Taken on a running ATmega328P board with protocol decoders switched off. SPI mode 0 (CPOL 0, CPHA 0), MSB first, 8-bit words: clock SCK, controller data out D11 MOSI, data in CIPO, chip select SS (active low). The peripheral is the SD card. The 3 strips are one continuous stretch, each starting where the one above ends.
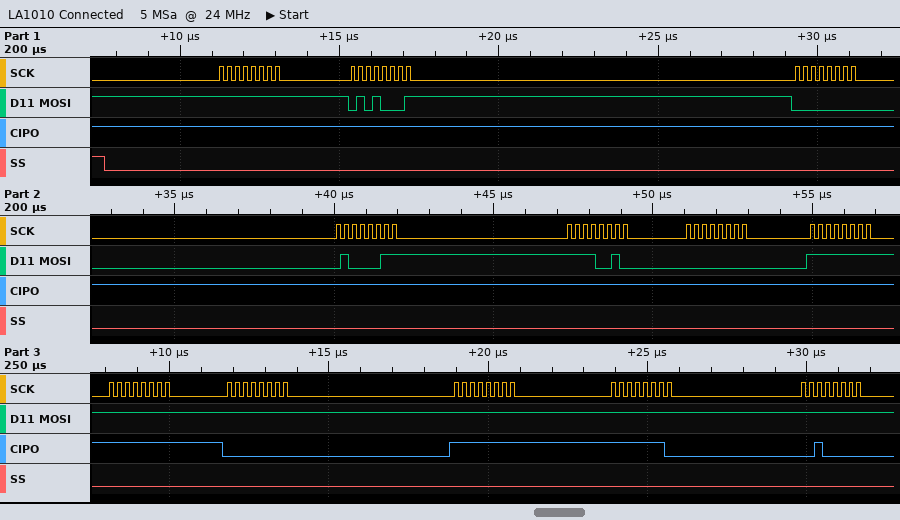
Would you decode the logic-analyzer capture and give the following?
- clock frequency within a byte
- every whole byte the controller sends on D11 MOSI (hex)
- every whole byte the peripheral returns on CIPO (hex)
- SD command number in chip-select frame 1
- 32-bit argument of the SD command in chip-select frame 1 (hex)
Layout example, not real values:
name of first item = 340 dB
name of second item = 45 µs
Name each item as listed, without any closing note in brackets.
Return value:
clock frequency within a byte = 4 MHz
every whole byte the controller sends on D11 MOSI = FF 51 00 43 F2 00 FF FF FF FF FF FF
every whole byte the peripheral returns on CIPO = FF FF FF FF FF FF FF FF 00 FF FE 20
SD command number in chip-select frame 1 = CMD17
32-bit argument of the SD command in chip-select frame 1 = 0x0043F200
